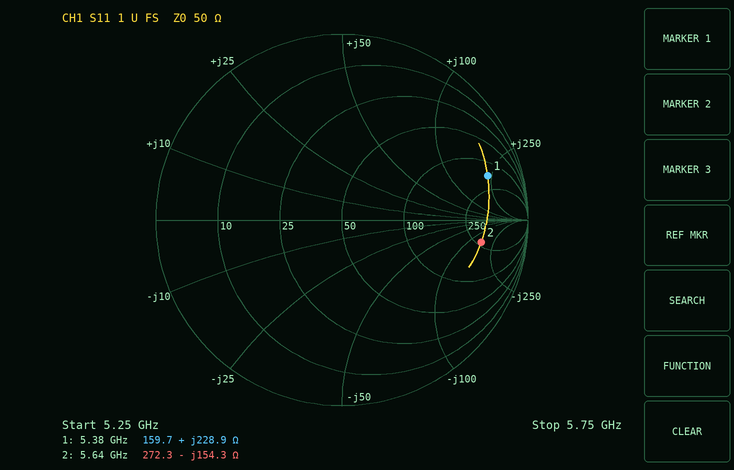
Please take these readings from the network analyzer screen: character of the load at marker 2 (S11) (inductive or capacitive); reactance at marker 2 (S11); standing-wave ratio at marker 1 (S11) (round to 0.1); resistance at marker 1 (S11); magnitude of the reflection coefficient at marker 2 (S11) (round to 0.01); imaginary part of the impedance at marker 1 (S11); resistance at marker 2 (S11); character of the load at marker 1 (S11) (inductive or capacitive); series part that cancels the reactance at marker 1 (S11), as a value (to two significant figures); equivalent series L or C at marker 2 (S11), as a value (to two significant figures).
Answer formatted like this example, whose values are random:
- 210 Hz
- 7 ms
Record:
- capacitive
- -154.3 Ω
- 10.0
- 159.7 Ω
- 0.76
- +228.9 Ω
- 272.3 Ω
- inductive
- 130 fF
- 180 fF
